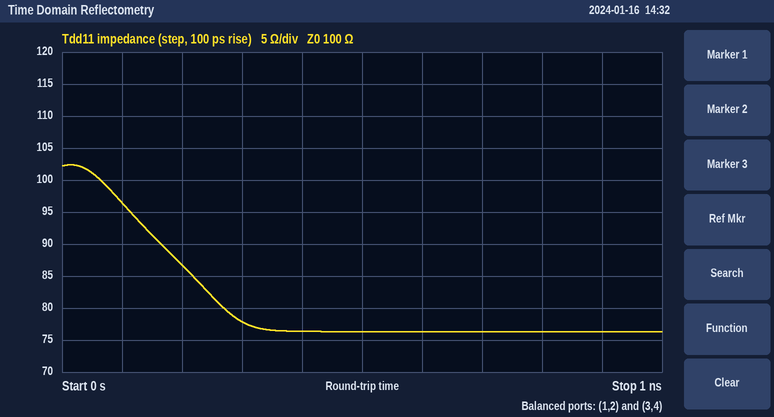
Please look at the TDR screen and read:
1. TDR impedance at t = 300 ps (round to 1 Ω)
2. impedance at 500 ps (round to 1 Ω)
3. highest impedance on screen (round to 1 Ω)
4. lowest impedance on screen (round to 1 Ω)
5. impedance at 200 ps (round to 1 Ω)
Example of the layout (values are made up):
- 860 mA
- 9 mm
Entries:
- 78 Ω
- 76 Ω
- 102 Ω
- 76 Ω
- 87 Ω
